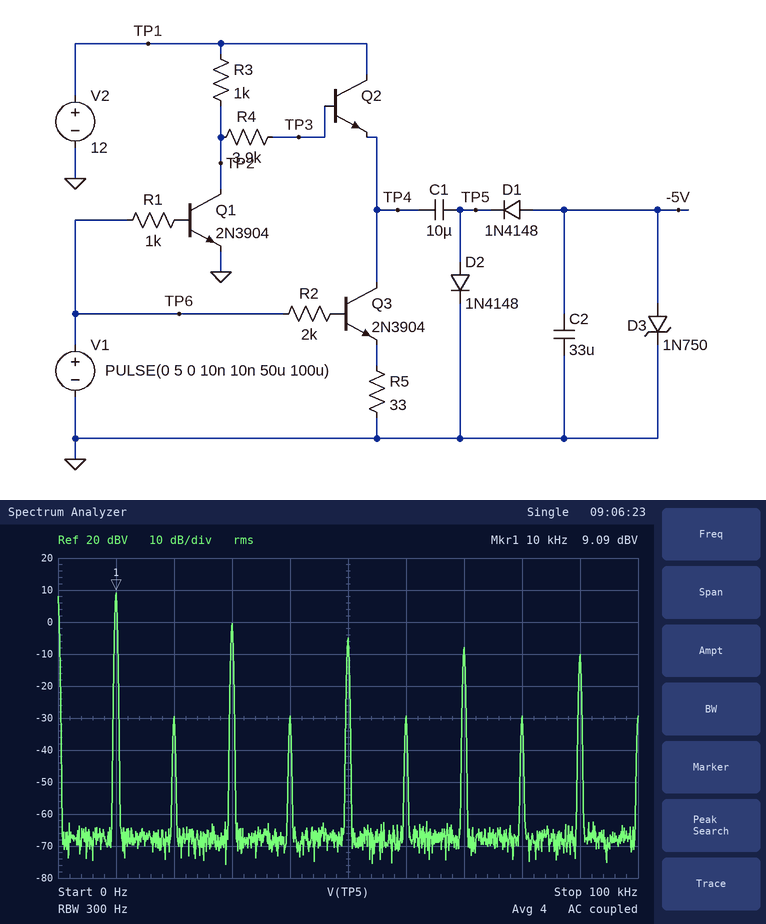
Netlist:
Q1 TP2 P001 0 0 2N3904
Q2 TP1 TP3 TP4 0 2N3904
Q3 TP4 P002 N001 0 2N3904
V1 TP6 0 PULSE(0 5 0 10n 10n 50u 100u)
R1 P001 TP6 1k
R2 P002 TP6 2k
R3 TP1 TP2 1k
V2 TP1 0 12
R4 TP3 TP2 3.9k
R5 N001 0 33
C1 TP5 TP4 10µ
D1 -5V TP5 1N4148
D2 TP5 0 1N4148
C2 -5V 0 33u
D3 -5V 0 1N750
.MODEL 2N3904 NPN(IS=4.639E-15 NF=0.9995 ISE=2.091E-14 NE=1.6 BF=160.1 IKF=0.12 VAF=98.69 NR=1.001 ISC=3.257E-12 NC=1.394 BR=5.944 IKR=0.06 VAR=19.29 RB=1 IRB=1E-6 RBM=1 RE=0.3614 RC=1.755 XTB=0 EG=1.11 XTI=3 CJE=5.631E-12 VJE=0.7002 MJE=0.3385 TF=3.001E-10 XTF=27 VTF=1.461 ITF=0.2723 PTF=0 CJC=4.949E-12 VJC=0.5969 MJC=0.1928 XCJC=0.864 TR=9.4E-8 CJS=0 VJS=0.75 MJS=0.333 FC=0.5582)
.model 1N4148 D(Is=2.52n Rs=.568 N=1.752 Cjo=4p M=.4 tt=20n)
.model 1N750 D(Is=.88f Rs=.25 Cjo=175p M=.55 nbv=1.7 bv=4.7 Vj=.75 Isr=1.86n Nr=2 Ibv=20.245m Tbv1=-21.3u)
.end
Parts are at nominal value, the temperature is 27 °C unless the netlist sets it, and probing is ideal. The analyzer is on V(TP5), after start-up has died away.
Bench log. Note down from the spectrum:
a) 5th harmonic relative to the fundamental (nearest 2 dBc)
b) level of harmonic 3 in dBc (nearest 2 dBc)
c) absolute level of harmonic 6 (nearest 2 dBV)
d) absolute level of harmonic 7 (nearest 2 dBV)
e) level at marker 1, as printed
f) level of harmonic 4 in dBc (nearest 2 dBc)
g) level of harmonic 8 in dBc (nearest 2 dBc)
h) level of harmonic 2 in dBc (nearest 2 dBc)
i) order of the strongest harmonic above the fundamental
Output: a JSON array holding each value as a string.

["-14 dBc", "-10 dBc", "-30 dBV", "-8 dBV", "9.09 dBV", "-38 dBc", "-38 dBc", "-38 dBc", "3"]
